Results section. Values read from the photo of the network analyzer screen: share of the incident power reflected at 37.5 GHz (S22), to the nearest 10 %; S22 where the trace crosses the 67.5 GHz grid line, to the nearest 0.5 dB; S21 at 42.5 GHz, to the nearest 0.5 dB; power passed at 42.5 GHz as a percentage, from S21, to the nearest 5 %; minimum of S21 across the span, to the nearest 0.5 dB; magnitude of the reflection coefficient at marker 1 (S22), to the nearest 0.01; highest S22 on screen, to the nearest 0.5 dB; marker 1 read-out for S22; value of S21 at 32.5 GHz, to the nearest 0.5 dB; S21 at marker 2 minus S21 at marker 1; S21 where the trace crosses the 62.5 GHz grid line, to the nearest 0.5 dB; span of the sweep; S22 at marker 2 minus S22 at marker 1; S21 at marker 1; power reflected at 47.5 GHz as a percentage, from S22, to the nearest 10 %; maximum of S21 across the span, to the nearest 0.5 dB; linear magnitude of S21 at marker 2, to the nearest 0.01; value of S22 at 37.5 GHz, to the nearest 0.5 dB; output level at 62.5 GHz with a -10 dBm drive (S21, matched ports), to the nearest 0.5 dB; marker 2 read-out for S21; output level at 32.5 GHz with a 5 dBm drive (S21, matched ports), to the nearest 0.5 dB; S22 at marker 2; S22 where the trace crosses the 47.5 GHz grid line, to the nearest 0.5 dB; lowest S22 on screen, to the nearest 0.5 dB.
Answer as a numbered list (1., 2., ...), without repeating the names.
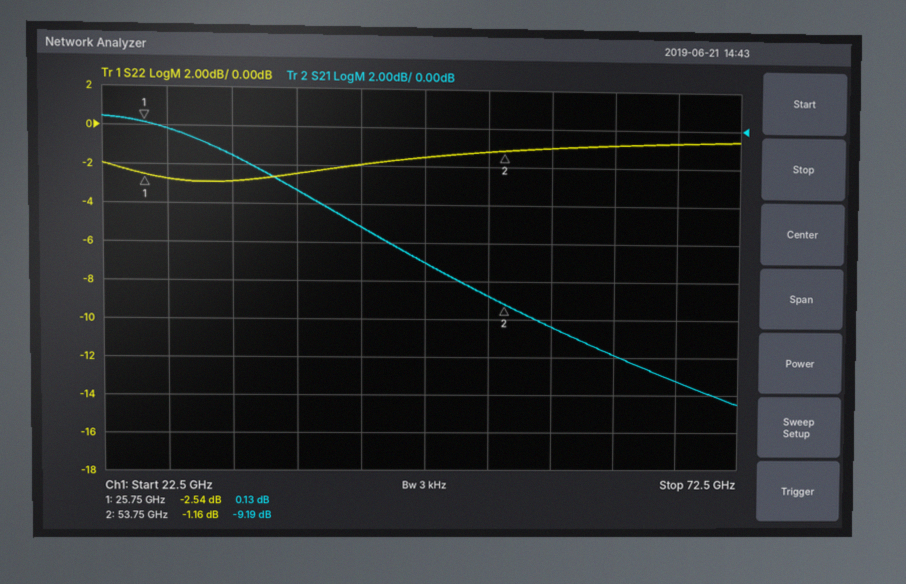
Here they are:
1. 60 %
2. -0.5 dB
3. -5.0 dB
4. 30 %
5. -14.5 dB
6. 0.75
7. -0.5 dB
8. -2.54 dB
9. -1.5 dB
10. -9.32 dB
11. -12.0 dB
12. 50 GHz
13. 1.38 dB
14. 0.13 dB
15. 70 %
16. 0.5 dB
17. 0.35
18. -2.5 dB
19. -22.0 dBm
20. -9.19 dB
21. 3.5 dBm
22. -1.16 dB
23. -1.5 dB
24. -3.0 dB
